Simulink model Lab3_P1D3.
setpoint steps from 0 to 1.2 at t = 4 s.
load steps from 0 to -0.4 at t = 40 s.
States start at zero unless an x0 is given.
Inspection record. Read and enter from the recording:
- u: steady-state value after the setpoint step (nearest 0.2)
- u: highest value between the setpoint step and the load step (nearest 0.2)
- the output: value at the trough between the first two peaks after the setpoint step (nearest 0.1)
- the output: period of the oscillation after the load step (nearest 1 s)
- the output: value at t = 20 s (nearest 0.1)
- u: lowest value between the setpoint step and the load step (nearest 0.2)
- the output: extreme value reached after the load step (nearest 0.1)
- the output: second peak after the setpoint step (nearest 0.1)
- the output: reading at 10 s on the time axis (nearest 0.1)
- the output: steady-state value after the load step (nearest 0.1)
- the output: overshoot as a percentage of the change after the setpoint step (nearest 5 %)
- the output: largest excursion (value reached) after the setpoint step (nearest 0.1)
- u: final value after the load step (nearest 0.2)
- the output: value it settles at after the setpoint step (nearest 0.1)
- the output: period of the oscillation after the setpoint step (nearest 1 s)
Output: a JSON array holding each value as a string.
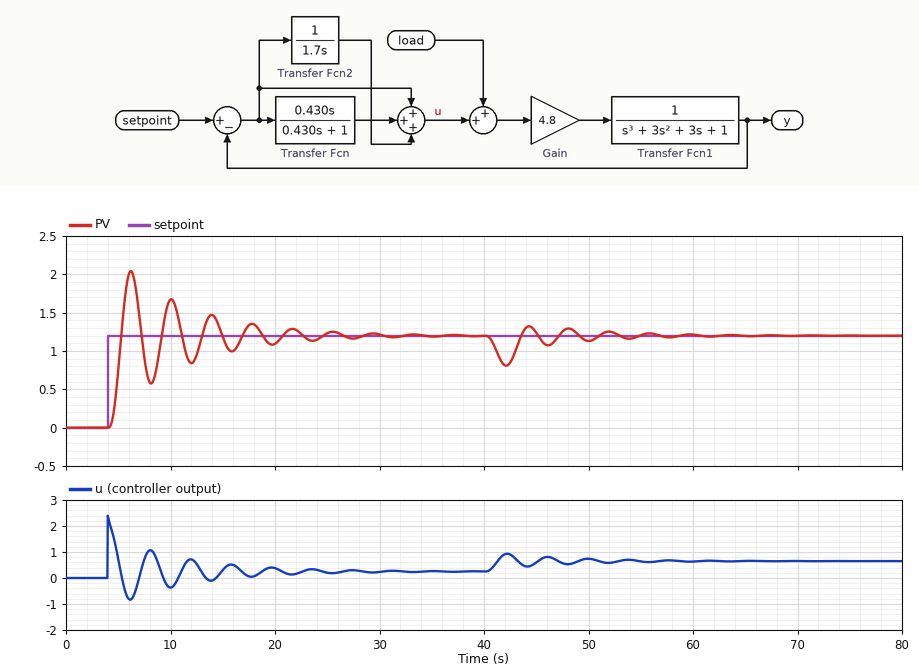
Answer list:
["0.2", "2.4", "0.6", "4 s", "1.1", "-0.8", "0.8", "1.7", "1.7", "1.2", "70 %", "2.0", "0.6", "1.2", "4 s"]
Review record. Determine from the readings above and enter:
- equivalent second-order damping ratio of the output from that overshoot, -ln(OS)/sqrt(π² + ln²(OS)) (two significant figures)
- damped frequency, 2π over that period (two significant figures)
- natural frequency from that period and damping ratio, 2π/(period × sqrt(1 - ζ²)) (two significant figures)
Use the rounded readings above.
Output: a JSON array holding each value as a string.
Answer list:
["0.11", "1.6 rad/s", "1.6 rad/s"]
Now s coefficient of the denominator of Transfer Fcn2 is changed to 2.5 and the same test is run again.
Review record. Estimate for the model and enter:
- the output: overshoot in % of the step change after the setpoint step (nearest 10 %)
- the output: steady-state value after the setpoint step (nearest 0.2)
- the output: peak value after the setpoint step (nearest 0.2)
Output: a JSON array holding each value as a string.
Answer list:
["60 %", "1.2", "1.8"]
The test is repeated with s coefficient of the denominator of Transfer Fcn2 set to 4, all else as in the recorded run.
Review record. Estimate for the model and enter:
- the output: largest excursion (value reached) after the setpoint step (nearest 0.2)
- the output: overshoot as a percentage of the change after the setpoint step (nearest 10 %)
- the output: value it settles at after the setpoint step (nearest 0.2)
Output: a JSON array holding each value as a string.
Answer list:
["1.8", "50 %", "1.2"]
